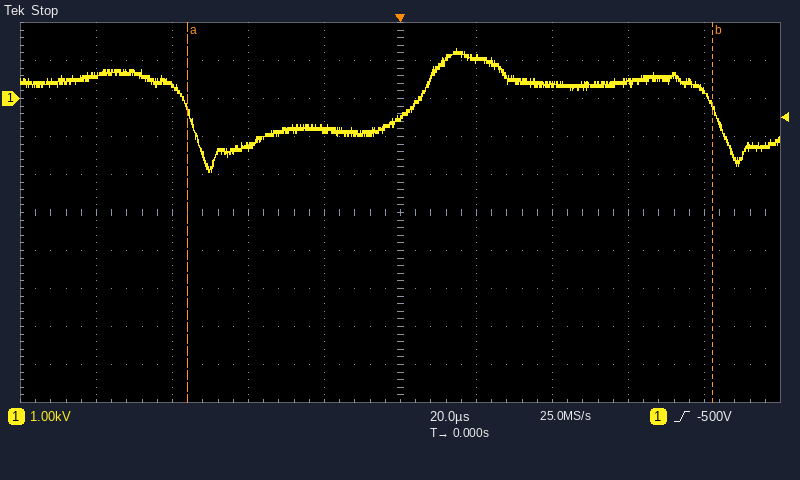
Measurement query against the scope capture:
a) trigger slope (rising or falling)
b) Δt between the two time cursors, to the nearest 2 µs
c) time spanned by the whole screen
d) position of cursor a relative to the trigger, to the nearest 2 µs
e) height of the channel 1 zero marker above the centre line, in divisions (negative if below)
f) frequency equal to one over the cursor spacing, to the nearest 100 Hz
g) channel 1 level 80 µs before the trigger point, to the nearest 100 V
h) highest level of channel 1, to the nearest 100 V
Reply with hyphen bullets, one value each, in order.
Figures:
- rising
- 138 µs
- 200 µs
- -56 µs
- +3.0 div
- 7.2 kHz
- 600 V
- 1.3 kV
